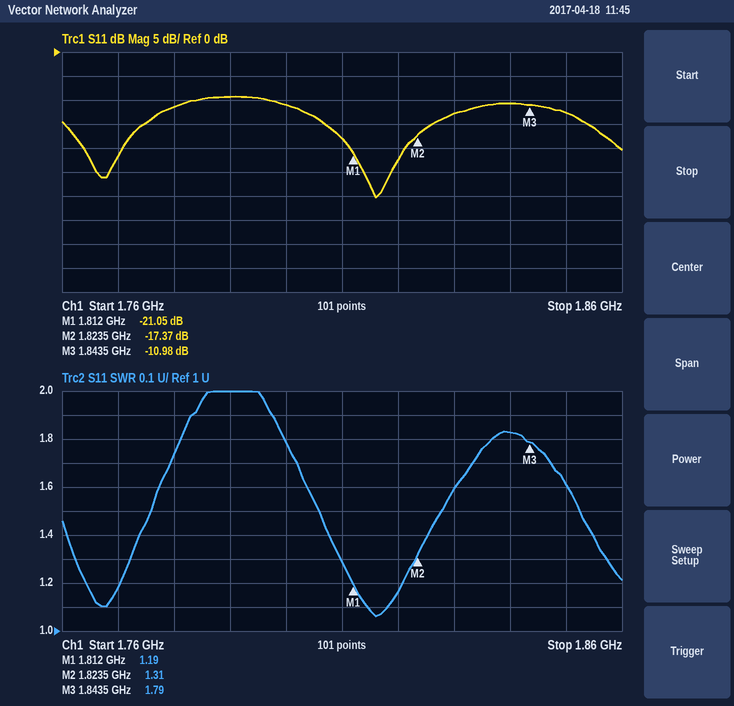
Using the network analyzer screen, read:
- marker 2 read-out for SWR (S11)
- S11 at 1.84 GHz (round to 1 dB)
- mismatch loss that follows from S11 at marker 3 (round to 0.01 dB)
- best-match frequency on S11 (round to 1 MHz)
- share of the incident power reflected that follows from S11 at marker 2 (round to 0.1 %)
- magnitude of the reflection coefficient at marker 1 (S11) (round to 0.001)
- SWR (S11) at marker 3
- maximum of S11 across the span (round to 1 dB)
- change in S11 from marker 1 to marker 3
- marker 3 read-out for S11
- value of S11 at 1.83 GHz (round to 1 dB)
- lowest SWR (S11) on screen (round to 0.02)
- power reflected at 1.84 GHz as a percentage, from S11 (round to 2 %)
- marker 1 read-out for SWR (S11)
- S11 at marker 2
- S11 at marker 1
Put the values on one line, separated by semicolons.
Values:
1.31; -11 dB; 0.36 dB; 1.816 GHz; 1.8 %; 0.089; 1.79; -9 dB; 10.07 dB; -10.98 dB; -13 dB; 1.06; 8 %; 1.19; -17.37 dB; -21.05 dB
